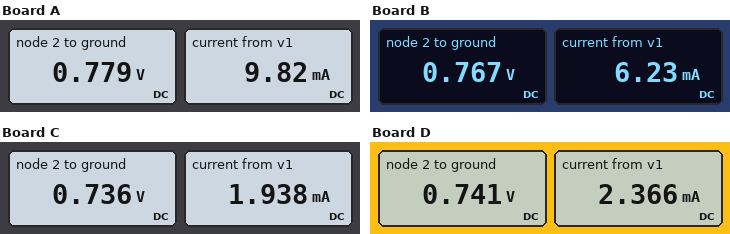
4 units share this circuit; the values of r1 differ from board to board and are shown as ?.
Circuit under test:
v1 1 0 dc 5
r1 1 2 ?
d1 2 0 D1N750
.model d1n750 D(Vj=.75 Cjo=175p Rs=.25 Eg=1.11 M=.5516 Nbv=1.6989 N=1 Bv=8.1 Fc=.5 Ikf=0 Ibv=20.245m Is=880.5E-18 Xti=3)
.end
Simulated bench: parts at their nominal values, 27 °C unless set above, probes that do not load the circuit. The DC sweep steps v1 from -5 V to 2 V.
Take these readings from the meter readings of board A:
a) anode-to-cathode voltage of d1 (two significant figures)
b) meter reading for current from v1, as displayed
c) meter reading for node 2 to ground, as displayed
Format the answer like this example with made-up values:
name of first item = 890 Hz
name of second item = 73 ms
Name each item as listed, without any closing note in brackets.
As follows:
anode-to-cathode voltage of d1 = 780 mV
meter reading for current from v1, as displayed = 9.82 mA
meter reading for node 2 to ground, as displayed = 0.779 V
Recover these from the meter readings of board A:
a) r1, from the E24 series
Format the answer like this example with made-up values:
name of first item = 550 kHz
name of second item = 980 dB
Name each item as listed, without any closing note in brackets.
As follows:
r1, from the E24 series = 430 Ω
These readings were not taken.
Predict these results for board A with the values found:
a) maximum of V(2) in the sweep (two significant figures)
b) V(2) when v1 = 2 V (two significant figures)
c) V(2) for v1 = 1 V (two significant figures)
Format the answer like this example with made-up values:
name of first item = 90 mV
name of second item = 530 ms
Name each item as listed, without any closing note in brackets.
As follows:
maximum of V(2) in the sweep = 750 mV
V(2) when v1 = 2 V = 750 mV
V(2) for v1 = 1 V = 710 mV
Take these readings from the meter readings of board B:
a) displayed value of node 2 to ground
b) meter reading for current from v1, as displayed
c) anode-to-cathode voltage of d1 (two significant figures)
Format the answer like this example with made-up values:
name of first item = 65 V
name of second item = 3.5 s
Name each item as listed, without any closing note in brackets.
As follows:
displayed value of node 2 to ground = 0.767 V
meter reading for current from v1, as displayed = 6.23 mA
anode-to-cathode voltage of d1 = 770 mV
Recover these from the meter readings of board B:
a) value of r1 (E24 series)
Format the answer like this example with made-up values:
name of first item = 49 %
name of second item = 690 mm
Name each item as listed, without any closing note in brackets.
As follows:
value of r1 = 680 Ω
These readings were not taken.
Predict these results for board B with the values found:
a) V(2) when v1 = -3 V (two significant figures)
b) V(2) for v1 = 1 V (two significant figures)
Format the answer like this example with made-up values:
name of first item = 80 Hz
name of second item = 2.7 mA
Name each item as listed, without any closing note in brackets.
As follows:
V(2) when v1 = -3 V = -3.0 V
V(2) for v1 = 1 V = 700 mV
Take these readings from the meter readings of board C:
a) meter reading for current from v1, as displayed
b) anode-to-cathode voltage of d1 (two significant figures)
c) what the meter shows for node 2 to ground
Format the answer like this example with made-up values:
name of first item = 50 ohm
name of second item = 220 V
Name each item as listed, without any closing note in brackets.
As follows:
meter reading for current from v1, as displayed = 1.938 mA
anode-to-cathode voltage of d1 = 740 mV
what the meter shows for node 2 to ground = 0.736 V
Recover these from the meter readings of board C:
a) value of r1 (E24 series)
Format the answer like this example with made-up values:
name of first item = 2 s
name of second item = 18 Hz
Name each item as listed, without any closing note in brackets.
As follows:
value of r1 = 2.2 kΩ
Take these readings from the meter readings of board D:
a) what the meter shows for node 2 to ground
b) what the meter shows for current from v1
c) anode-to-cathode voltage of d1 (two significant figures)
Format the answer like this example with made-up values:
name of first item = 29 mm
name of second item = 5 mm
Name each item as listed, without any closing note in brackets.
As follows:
what the meter shows for node 2 to ground = 0.741 V
what the meter shows for current from v1 = 2.366 mA
anode-to-cathode voltage of d1 = 740 mV
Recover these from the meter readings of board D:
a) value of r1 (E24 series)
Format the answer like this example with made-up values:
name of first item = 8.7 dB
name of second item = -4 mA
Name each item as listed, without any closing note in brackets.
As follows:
value of r1 = 1.8 kΩ
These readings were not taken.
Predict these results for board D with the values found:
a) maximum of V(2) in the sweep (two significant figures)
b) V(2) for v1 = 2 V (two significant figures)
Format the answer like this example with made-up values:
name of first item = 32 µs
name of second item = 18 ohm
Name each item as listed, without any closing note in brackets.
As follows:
maximum of V(2) in the sweep = 710 mV
V(2) for v1 = 2 V = 710 mV
